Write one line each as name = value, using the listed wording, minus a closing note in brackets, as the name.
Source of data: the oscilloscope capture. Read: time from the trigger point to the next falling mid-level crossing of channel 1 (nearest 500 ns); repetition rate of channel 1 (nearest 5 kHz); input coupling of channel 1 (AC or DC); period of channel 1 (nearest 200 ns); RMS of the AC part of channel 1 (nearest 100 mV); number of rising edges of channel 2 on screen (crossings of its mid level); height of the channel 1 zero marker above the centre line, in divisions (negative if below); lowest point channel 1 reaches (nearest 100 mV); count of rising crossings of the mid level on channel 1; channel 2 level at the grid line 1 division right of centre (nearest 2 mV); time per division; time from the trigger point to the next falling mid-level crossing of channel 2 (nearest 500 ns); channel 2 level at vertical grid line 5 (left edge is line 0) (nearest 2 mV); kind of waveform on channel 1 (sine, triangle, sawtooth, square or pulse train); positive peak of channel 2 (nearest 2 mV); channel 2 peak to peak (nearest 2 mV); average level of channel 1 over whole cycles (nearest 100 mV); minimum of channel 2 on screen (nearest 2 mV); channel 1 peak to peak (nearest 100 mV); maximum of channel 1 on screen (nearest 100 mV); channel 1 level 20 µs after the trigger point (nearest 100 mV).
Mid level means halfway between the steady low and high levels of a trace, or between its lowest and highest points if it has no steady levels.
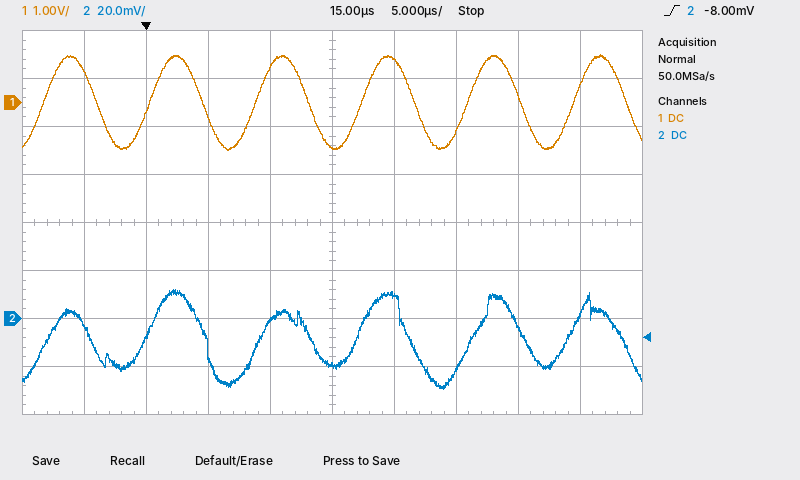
time from the trigger point to the next falling mid-level crossing of channel 1 = 4.5 µs
repetition rate of channel 1 = 115 kHz
input coupling of channel 1 = DC
period of channel 1 = 8.6 µs
RMS of the AC part of channel 1 = 700 mV
number of rising edges of channel 2 on screen = 6
height of the channel 1 zero marker above the centre line, in divisions = +2.5 div
lowest point channel 1 reaches = -1.0 V
count of rising crossings of the mid level on channel 1 = 6
channel 2 level at the grid line 1 division right of centre = 10 mV
time per division = 5 µs
time from the trigger point to the next falling mid-level crossing of channel 2 = 5.0 µs
channel 2 level at vertical grid line 5 (left edge is line 0) = -20 mV
kind of waveform on channel 1 = sine
positive peak of channel 2 = 12 mV
channel 2 peak to peak = 42 mV
average level of channel 1 over whole cycles = 0.0 V
minimum of channel 2 on screen = -30 mV
channel 1 peak to peak = 2.0 V
maximum of channel 1 on screen = 1.0 V
channel 1 level 20 µs after the trigger point = 900 mV
